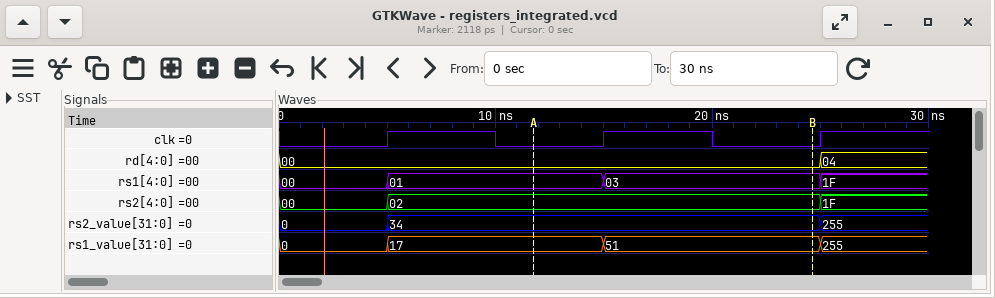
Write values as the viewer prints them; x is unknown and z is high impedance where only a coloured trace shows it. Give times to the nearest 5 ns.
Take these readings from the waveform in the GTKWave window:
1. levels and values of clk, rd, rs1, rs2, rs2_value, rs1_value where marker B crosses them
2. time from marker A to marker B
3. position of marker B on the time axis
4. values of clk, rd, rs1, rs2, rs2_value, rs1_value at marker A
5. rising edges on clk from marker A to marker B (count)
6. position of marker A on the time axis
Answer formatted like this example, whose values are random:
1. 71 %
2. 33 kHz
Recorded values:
1. clk=0, rd=00, rs1=03, rs2=02, rs2_value=34, rs1_value=51
2. 15 ns
3. 25 ns
4. clk=0, rd=00, rs1=01, rs2=02, rs2_value=34, rs1_value=17
5. 1
6. 10 ns
